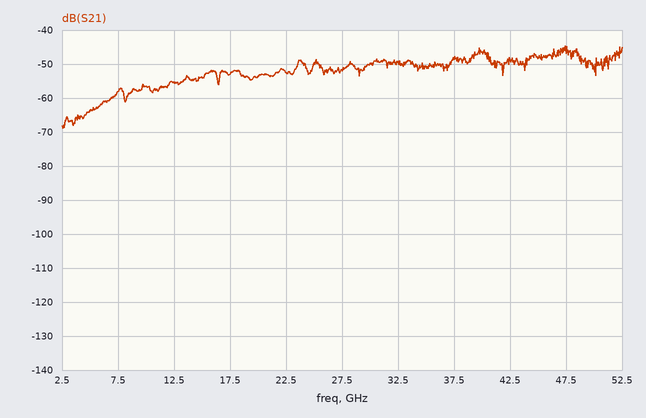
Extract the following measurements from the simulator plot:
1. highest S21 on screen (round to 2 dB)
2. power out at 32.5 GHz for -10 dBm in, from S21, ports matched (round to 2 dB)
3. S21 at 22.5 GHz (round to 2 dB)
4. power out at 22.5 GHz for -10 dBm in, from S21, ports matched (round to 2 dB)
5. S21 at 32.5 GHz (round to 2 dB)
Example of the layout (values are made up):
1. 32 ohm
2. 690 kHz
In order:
1. -44 dB
2. -60 dBm
3. -52 dB
4. -62 dBm
5. -50 dB
